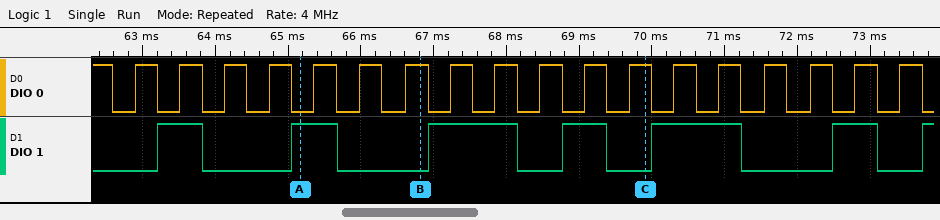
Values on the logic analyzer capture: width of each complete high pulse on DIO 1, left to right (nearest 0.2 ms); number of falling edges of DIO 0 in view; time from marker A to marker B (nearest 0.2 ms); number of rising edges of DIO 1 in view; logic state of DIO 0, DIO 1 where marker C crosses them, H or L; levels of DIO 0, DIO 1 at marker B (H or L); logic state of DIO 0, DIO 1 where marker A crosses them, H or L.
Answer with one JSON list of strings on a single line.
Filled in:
["0.6 ms, 0.6 ms, 1.2 ms, 0.6 ms, 1.2 ms, 0.6 ms", "19", "1.6 ms", "7", "DIO 0=H, DIO 1=L", "DIO 0=H, DIO 1=L", "DIO 0=L, DIO 1=H"]
